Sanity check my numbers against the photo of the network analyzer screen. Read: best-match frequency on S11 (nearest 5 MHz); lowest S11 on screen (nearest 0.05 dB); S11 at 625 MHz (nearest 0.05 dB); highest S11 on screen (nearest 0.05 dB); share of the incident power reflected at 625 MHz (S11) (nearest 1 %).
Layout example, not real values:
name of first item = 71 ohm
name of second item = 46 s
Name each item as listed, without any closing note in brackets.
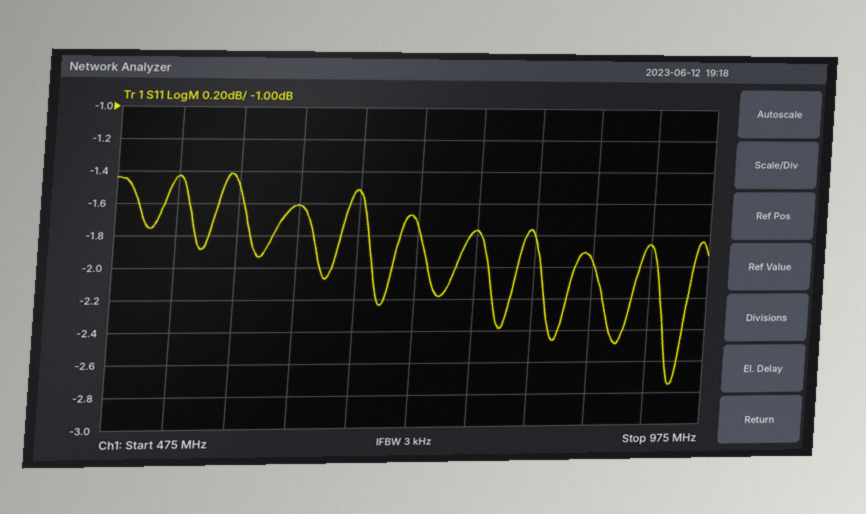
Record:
best-match frequency on S11 = 945 MHz
lowest S11 on screen = -2.75 dB
S11 at 625 MHz = -1.60 dB
highest S11 on screen = -1.40 dB
share of the incident power reflected at 625 MHz (S11) = 69 %
